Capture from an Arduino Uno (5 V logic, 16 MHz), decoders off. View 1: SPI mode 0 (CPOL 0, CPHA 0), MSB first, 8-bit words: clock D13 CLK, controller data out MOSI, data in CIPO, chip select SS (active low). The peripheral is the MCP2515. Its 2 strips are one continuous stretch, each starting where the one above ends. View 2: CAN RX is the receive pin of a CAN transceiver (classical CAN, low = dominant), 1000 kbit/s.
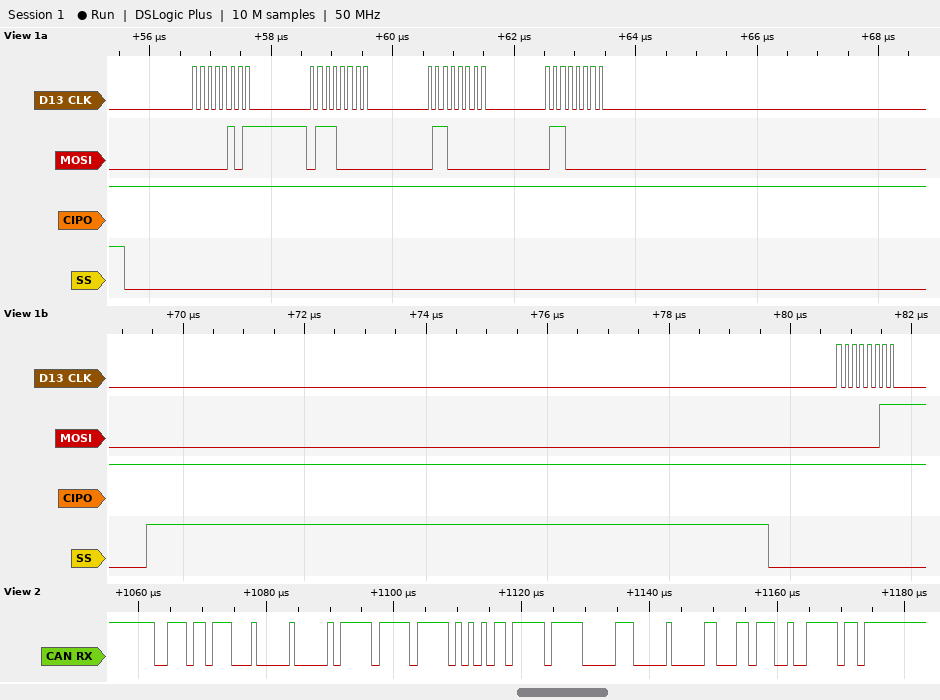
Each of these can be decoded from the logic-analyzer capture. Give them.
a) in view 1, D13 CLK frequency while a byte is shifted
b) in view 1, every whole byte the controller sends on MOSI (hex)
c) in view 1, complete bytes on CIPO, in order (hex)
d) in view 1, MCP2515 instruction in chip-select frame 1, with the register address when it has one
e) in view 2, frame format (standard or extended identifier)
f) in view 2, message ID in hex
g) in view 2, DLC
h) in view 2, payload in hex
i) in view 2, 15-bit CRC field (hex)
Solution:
8 MHz
05 70 60 60 03
FF FF FF FF FF
BIT MODIFY 0x70
standard
0x3B7
8
00 FF FF 56 FF C3 00 23
0x393F
